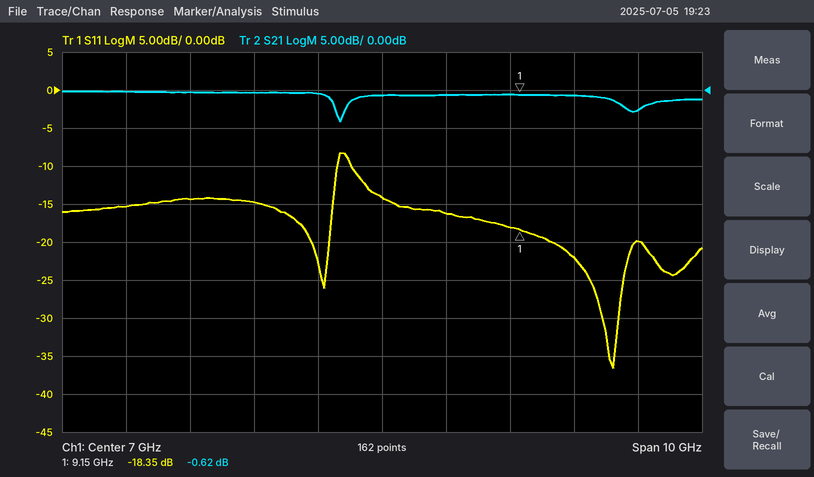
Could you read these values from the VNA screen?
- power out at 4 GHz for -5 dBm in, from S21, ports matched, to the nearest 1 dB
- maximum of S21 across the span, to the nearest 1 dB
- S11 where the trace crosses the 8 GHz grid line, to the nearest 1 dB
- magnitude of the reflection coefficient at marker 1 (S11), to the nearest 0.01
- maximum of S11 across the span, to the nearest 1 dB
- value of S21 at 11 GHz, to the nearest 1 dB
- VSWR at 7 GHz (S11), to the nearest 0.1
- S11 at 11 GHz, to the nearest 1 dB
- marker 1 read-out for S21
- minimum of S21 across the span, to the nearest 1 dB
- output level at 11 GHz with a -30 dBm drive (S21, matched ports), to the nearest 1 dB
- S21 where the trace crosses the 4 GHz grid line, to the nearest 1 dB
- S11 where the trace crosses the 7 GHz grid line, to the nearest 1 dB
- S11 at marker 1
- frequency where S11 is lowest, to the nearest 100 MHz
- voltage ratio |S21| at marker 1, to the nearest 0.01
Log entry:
-5 dBm
0 dB
-16 dB
0.12
-8 dB
-3 dB
1.5
-20 dB
-0.62 dB
-4 dB
-33 dBm
0 dB
-14 dB
-18.35 dB
10.6 GHz
0.93
